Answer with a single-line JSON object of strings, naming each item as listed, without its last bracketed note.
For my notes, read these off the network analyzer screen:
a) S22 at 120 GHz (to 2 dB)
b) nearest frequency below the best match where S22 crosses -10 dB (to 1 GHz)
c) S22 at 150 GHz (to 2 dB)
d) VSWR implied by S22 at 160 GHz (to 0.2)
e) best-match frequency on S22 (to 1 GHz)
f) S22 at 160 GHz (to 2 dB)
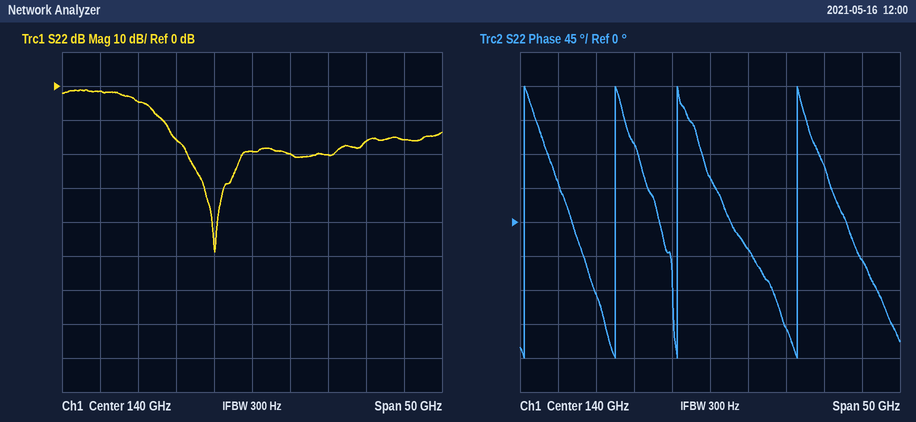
{"S22 at 120 GHz": "-2 dB", "nearest frequency below the best match where S22 crosses -10 dB": "128 GHz", "S22 at 150 GHz": "-20 dB", "VSWR implied by S22 at 160 GHz": "1.4", "best-match frequency on S22": "135 GHz", "S22 at 160 GHz": "-16 dB"}
